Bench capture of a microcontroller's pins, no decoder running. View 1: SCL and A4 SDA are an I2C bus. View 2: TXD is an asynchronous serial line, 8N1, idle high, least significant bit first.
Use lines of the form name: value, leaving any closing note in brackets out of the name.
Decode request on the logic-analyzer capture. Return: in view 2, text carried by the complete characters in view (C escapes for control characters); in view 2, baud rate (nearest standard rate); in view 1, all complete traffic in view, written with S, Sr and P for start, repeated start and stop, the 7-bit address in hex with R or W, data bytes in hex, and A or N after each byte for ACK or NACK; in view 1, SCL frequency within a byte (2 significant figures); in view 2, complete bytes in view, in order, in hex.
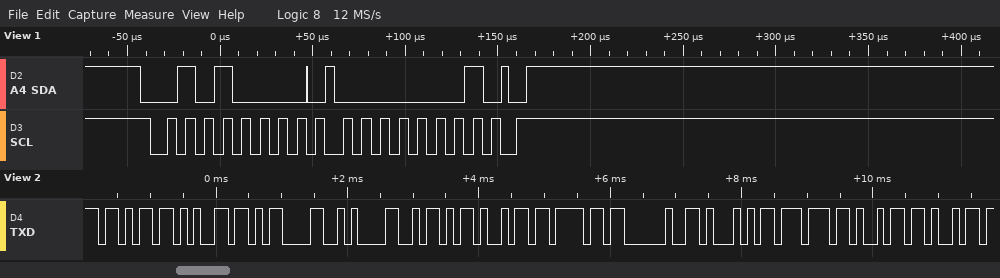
in view 2, text carried by the complete characters in view: "ke\r\nZio Qwii"
in view 2, baud rate: 9600 baud
in view 1, all complete traffic in view, written with S, Sr and P for start, repeated start and stop, the 7-bit address in hex with R or W, data bytes in hex, and A or N after each byte for ACK or NACK: S 28W A 01 A P
in view 1, SCL frequency within a byte: 100 kHz
in view 2, complete bytes in view, in order, in hex: 0x6B 0x65 0x0D 0x0A 0x5A 0x69 0x6F 0x20 0x51 0x77 0x69 0x69
